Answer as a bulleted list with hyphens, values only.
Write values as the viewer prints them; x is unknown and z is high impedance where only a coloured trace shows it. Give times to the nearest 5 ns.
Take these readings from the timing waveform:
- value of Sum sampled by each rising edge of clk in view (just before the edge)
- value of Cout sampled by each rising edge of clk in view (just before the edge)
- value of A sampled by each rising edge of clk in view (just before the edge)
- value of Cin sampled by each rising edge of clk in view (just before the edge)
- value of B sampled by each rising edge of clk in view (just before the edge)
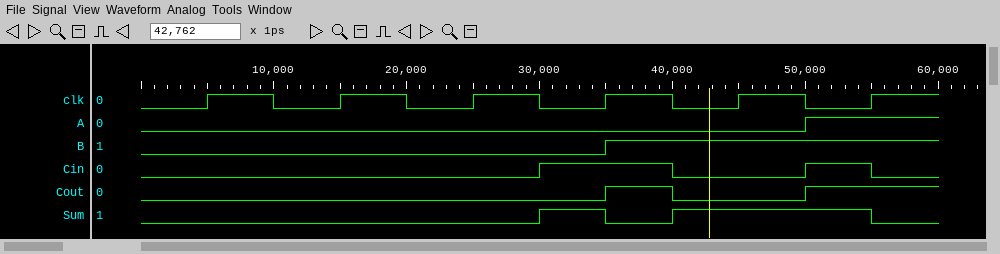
- 0 0 0 1 1 1
- 0 0 0 0 0 1
- 0 0 0 0 0 1
- 0 0 0 1 0 1
- 0 0 0 0 1 1
